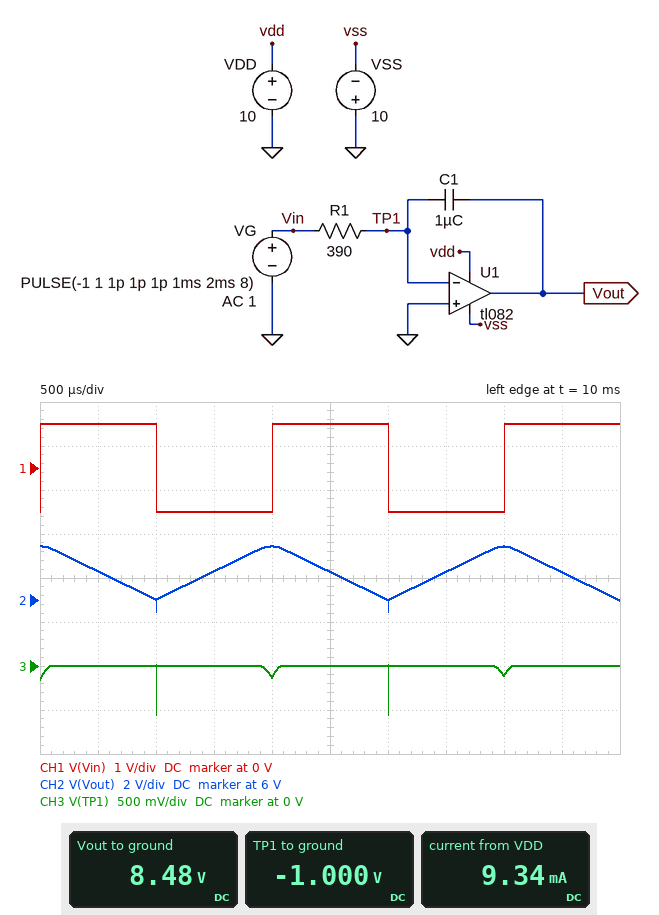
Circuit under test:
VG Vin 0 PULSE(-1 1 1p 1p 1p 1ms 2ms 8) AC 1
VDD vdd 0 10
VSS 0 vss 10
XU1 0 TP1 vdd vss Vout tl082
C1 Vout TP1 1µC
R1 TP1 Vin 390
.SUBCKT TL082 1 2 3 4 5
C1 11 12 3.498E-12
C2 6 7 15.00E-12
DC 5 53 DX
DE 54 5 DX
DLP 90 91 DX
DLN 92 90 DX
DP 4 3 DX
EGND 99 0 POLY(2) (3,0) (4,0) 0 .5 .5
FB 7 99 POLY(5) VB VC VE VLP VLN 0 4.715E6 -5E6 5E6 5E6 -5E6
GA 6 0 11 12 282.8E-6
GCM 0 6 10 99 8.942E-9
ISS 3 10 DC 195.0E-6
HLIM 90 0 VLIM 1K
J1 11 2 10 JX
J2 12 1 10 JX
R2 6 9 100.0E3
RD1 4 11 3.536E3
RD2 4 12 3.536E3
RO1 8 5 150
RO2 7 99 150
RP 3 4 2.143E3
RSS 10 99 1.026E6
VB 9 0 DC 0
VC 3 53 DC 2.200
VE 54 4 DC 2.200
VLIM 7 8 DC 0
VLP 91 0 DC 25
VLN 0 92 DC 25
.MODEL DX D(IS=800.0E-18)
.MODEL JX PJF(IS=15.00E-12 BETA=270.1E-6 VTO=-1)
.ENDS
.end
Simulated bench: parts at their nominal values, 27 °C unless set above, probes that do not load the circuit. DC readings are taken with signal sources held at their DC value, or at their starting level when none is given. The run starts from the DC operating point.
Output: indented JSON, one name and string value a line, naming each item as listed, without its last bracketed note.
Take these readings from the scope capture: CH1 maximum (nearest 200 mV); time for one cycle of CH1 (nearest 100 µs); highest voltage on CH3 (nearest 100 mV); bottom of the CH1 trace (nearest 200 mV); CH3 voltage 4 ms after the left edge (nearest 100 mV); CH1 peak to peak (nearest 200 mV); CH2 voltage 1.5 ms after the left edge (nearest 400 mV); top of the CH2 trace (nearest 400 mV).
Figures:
{
  "CH1 maximum": "1.0 V",
  "time for one cycle of CH1": "2.0 ms",
  "highest voltage on CH3": "0 V",
  "bottom of the CH1 trace": "-1.0 V",
  "CH3 voltage 4 ms after the left edge": "-100 mV",
  "CH1 peak to peak": "2.0 V",
  "CH2 voltage 1.5 ms after the left edge": "7.2 V",
  "top of the CH2 trace": "8.4 V"
}
